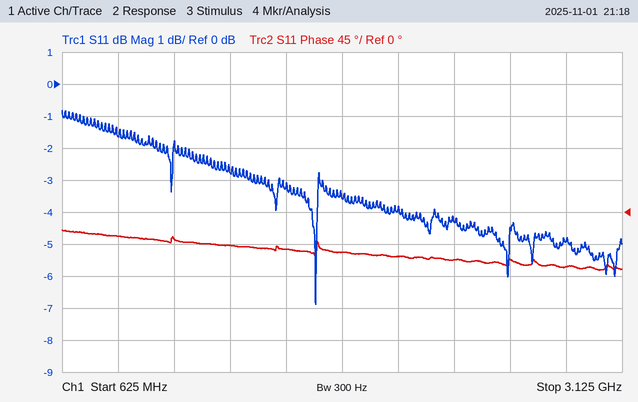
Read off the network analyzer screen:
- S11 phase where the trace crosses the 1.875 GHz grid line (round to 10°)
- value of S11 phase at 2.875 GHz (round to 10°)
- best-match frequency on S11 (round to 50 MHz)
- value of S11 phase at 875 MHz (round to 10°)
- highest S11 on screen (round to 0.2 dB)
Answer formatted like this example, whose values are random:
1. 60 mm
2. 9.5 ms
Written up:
1. -60°
2. -80°
3. 1.75 GHz
4. -30°
5. -0.8 dB
